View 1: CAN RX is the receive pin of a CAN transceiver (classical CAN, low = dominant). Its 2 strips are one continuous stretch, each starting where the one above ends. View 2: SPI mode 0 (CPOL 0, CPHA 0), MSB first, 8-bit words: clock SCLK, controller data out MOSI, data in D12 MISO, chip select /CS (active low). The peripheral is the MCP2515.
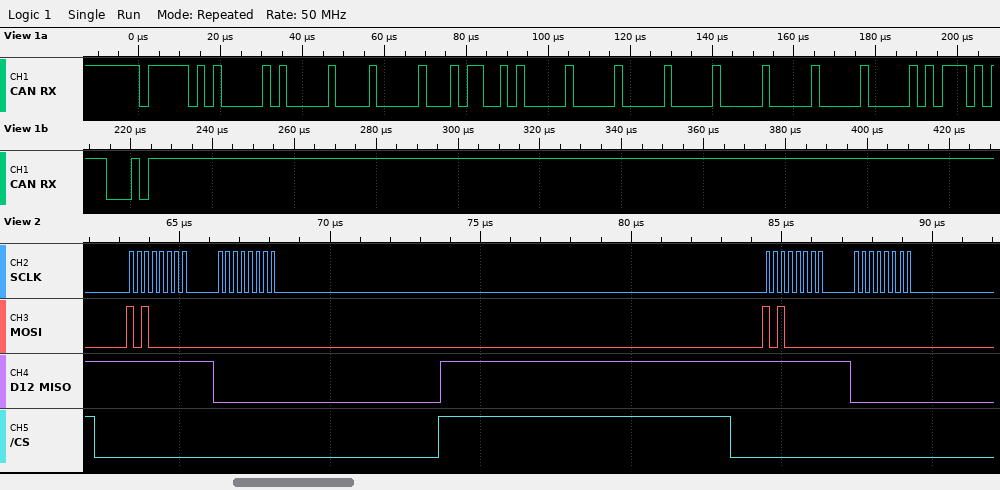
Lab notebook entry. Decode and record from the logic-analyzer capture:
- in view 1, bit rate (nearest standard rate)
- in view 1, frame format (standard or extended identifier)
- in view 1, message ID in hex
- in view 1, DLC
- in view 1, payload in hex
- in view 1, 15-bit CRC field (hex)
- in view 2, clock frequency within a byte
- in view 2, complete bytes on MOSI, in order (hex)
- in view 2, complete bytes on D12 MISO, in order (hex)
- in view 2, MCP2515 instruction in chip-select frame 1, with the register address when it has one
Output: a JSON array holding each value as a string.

["500 kbit/s", "standard", "0x7E8", "8", "02 01 65 00 00 00 00 00", "0x2EB8", "4 MHz", "0xA0 0x00 0xA0 0x00", "0xFF 0x00 0xFF 0x00", "READ STATUS"]
